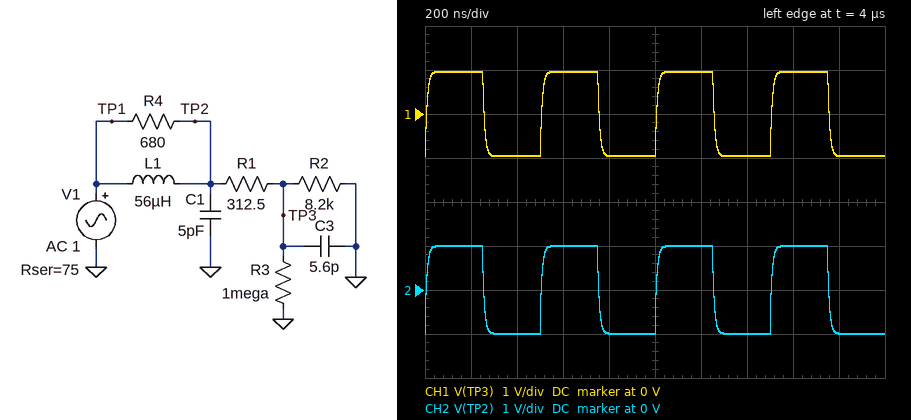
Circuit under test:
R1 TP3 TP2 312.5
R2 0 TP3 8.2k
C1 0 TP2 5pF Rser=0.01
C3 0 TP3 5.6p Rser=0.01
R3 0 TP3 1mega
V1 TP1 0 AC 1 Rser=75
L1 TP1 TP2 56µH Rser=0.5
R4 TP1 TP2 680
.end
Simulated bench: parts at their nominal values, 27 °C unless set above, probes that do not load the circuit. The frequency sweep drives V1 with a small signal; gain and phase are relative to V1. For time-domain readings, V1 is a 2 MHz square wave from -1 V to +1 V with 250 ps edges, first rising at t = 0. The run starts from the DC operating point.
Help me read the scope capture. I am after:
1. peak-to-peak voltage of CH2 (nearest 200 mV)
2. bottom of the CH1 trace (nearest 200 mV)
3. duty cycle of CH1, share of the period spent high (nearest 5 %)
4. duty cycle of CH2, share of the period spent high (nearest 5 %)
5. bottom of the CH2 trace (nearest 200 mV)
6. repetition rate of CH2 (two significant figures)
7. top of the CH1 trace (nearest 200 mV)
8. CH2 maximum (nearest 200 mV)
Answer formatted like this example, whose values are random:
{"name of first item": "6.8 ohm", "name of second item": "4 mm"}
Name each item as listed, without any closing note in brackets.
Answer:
{"peak-to-peak voltage of CH2": "2.0 V", "bottom of the CH1 trace": "-1.0 V", "duty cycle of CH1, share of the period spent high": "50 %", "duty cycle of CH2, share of the period spent high": "50 %", "bottom of the CH2 trace": "-1.0 V", "repetition rate of CH2": "2.0 MHz", "top of the CH1 trace": "1.0 V", "CH2 maximum": "1.0 V"}
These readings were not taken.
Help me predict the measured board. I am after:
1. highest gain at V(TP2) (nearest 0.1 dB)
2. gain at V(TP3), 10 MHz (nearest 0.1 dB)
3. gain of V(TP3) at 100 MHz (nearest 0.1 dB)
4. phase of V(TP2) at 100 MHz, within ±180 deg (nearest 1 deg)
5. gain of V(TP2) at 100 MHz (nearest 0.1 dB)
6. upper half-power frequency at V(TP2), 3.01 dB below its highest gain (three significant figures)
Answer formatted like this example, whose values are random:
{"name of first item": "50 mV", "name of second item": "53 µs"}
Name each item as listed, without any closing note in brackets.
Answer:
{"highest gain at V(TP2)": "-0.1 dB", "gain at V(TP3), 10 MHz": "-1.5 dB", "gain of V(TP3) at 100 MHz": "-16.1 dB", "phase of V(TP2) at 100 MHz, within ±180 deg": "-58 deg", "gain of V(TP2) at 100 MHz": "-12.5 dB", "upper half-power frequency at V(TP2), 3.01 dB below its highest gain": "19.1 MHz"}
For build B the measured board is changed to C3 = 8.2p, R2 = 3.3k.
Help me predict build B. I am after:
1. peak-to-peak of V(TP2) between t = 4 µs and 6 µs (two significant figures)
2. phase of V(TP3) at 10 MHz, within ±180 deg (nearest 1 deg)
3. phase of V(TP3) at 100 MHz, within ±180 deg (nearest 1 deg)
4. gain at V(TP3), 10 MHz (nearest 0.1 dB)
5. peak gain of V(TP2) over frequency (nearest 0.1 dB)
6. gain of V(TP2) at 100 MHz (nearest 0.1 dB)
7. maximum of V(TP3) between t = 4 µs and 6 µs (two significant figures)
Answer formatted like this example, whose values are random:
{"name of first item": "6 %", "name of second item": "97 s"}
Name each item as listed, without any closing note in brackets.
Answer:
{"peak-to-peak of V(TP2) between t = 4 µs and 6 µs": "1.9 V", "phase of V(TP3) at 10 MHz, within ±180 deg": "-35 deg", "phase of V(TP3) at 100 MHz, within ±180 deg": "-108 deg", "gain at V(TP3), 10 MHz": "-3.1 dB", "peak gain of V(TP2) over frequency": "-0.2 dB", "gain of V(TP2) at 100 MHz": "-12.7 dB", "maximum of V(TP3) between t = 4 µs and 6 µs": "880 mV"}
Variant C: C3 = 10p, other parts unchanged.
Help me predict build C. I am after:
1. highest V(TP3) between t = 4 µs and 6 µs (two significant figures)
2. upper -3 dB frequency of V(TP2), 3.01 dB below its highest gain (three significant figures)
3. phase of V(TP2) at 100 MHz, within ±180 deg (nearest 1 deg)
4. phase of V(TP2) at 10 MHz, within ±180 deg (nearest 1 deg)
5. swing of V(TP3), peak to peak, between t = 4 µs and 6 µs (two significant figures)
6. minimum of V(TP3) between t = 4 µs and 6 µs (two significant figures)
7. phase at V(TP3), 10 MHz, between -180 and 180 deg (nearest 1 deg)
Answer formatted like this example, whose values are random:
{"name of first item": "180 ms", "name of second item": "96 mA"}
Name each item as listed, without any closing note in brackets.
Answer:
{"highest V(TP3) between t = 4 µs and 6 µs": "990 mV", "upper -3 dB frequency of V(TP2), 3.01 dB below its highest gain": "13.2 MHz", "phase of V(TP2) at 100 MHz, within ±180 deg": "-50 deg", "phase of V(TP2) at 10 MHz, within ±180 deg": "-32 deg", "swing of V(TP3), peak to peak, between t = 4 µs and 6 µs": "2.0 V", "minimum of V(TP3) between t = 4 µs and 6 µs": "-990 mV", "phase at V(TP3), 10 MHz, between -180 and 180 deg": "-43 deg"}
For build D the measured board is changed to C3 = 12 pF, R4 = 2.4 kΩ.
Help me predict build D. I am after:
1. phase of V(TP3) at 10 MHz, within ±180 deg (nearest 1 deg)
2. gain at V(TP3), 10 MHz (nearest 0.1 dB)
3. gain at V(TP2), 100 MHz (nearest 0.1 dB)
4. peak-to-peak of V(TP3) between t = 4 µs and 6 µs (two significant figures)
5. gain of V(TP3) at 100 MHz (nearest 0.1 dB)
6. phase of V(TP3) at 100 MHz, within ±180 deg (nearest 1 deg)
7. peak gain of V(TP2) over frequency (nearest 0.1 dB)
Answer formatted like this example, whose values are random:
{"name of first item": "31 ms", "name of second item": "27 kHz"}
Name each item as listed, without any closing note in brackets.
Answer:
{"phase of V(TP3) at 10 MHz, within ±180 deg": "-92 deg", "gain at V(TP3), 10 MHz": "-6.6 dB", "gain at V(TP2), 100 MHz": "-22.3 dB", "peak-to-peak of V(TP3) between t = 4 µs and 6 µs": "2.7 V", "gain of V(TP3) at 100 MHz": "-30.5 dB", "phase of V(TP3) at 100 MHz, within ±180 deg": "-124 deg", "peak gain of V(TP2) over frequency": "1.9 dB"}
